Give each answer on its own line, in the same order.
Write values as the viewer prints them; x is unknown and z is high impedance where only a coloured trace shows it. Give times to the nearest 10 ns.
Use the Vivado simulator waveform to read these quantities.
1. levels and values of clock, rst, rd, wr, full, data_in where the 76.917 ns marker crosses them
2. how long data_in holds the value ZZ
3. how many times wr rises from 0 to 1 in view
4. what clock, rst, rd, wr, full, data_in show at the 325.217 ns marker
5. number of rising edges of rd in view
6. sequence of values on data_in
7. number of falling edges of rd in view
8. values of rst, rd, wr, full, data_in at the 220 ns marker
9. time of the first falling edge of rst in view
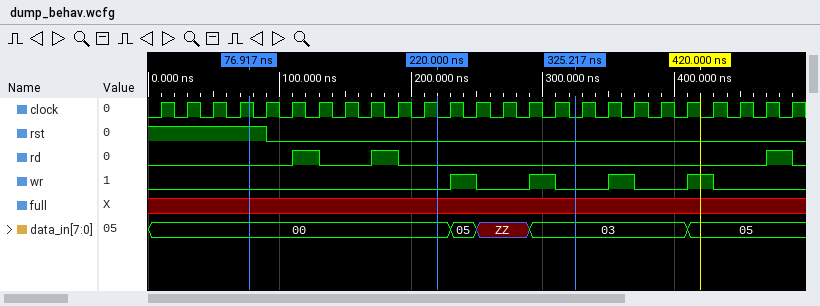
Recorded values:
clock=1, rst=1, rd=0, wr=0, full=x, data_in=00
40 ns
4
clock=0, rst=0, rd=0, wr=0, full=x, data_in=03
3
00, 05, ZZ, 03, 05
3
rst=0, rd=0, wr=0, full=x, data_in=00
90 ns
